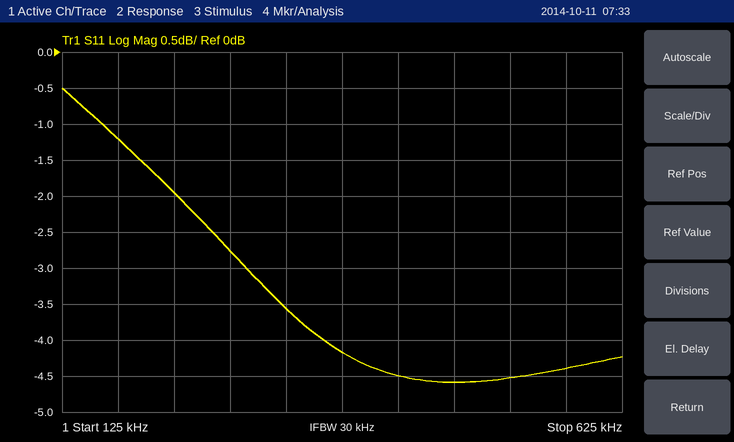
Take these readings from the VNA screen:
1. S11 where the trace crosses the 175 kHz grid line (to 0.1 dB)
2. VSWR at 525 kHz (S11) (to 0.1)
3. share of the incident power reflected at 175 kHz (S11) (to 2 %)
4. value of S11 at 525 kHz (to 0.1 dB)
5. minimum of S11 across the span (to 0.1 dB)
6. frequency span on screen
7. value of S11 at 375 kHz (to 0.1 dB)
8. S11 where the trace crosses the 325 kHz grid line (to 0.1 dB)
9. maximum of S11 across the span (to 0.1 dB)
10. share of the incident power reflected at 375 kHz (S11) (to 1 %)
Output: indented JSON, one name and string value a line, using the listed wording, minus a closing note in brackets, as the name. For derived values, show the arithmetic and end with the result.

{
  "S11 where the trace crosses the 175 kHz grid line": "-1.2 dB",
  "VSWR at 525 kHz (S11)": "|Γ| = 10^(-4.5/20) = 0.5957; VSWR = (1 + 0.5957)/(1 − 0.5957) ≈ 3.9",
  "share of the incident power reflected at 175 kHz (S11)": "10^(-1.2/10) ≈ 76 %",
  "value of S11 at 525 kHz": "-4.5 dB",
  "minimum of S11 across the span": "-4.6 dB",
  "frequency span on screen": "500 kHz",
  "value of S11 at 375 kHz": "-4.2 dB",
  "S11 where the trace crosses the 325 kHz grid line": "-3.6 dB",
  "maximum of S11 across the span": "-0.5 dB",
  "share of the incident power reflected at 375 kHz (S11)": "10^(-4.2/10) ≈ 38 %"
}
